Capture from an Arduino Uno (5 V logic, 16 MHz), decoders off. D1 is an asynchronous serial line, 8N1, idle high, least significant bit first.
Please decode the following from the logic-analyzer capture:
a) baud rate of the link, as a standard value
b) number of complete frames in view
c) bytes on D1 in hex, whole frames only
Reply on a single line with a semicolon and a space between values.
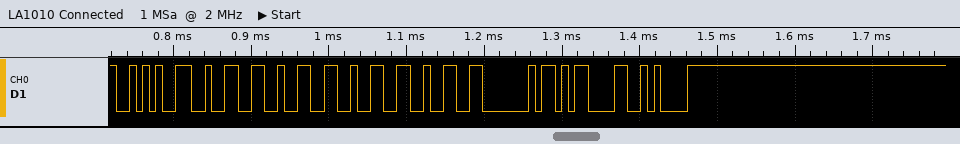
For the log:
115200 baud; 8; 0x2A 0x32 0x32 0x32 0x32 0x40 0x0D 0x0A
